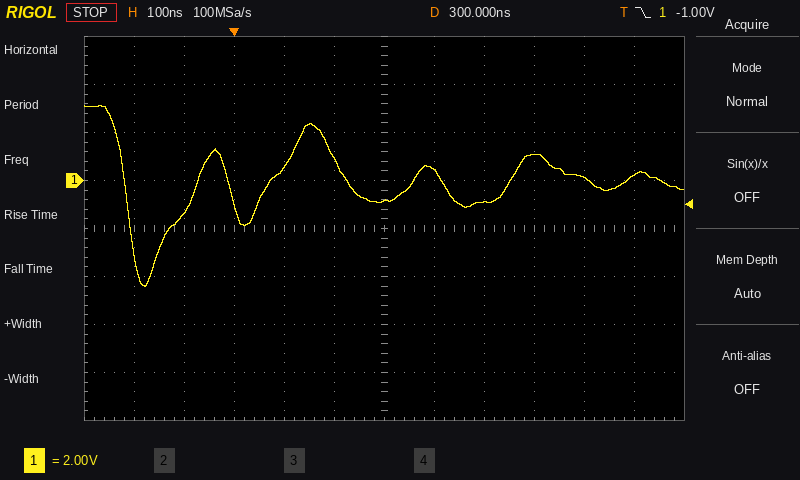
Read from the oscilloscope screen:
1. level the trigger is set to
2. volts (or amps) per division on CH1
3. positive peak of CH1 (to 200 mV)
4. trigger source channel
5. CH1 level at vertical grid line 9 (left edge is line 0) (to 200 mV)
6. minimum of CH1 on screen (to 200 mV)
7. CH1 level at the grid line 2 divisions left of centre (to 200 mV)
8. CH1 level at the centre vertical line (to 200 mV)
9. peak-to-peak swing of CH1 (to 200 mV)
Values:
-1.00 V
2 V
3.2 V
CH1
1.0 V
-4.4 V
600 mV
-800 mV
7.6 V
